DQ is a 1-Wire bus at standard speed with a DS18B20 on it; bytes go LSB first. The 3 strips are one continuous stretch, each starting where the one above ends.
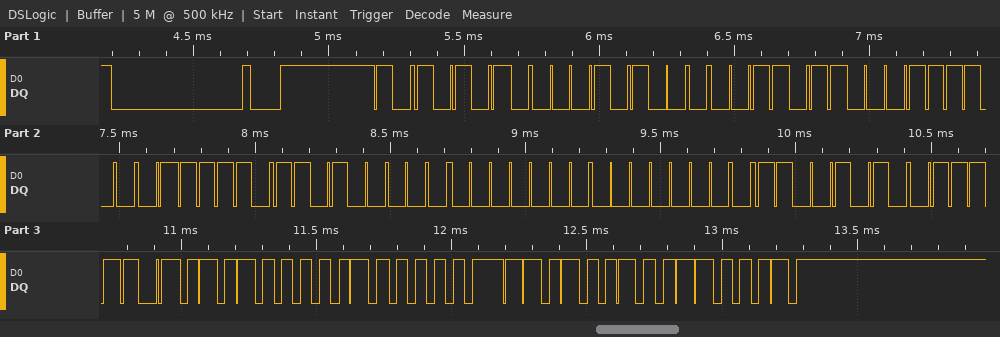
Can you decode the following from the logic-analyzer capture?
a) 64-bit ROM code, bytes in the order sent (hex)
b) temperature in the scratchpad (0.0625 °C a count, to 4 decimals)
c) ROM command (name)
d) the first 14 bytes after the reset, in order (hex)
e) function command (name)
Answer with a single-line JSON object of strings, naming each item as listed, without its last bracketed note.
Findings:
{"64-bit ROM code, bytes in the order sent": "28 D8 78 7C 0B 00 00 53", "temperature in the scratchpad": "32.6250 °C", "ROM command": "Match ROM", "the first 14 bytes after the reset, in order": "55 28 D8 78 7C 0B 00 00 53 BE 0A 02 4B 46", "function command": "Read Scratchpad"}
